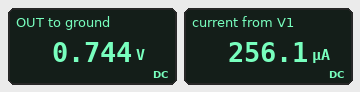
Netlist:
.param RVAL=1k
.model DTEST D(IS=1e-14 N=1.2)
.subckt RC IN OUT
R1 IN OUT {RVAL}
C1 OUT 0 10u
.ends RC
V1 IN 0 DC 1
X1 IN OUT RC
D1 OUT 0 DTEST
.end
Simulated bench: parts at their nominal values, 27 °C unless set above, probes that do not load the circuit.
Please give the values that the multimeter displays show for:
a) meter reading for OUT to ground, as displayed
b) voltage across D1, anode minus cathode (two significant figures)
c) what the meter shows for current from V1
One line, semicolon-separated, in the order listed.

0.744 V; 740 mV; 256.1 µA
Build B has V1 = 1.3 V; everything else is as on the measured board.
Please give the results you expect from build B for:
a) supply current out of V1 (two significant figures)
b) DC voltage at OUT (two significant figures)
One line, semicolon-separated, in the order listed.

530 µA; 770 mV
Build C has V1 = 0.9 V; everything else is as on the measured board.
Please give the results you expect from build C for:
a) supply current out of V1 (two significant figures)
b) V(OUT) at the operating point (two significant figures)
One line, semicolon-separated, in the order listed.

170 µA; 730 mV
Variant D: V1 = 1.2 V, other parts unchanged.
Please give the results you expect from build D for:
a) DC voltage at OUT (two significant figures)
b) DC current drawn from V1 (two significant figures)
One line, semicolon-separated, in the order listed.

760 mV; 440 µA
